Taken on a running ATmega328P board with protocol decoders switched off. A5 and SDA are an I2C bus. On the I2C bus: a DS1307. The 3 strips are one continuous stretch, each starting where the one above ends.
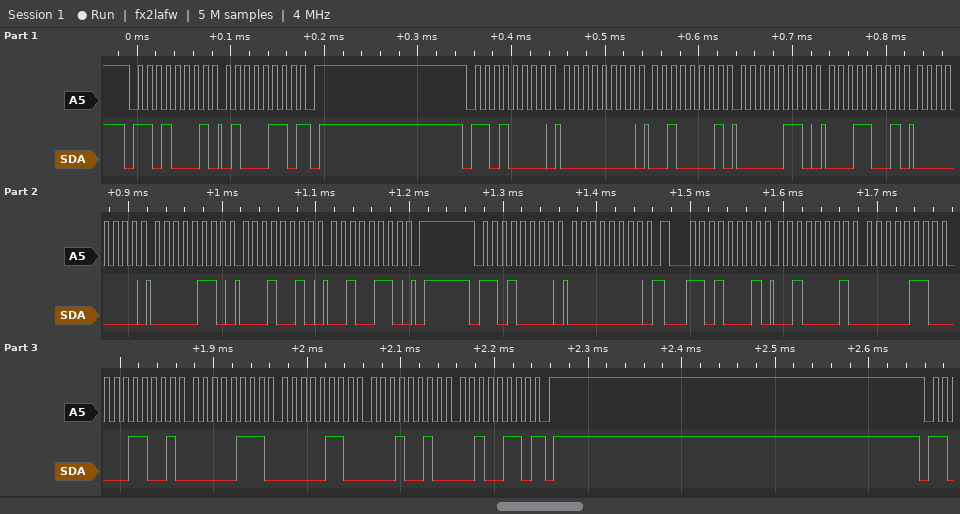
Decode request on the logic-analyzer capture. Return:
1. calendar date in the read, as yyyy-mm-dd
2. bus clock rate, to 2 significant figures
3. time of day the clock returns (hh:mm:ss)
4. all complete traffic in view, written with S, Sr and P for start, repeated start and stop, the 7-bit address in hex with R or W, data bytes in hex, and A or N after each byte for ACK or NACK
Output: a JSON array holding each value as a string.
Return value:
["2026-12-06", "100 kHz", "19:06:21", "S 68R A 46 N P S 68W A 00 A 21 A 06 A 19 A 00 A 06 A 12 A 26 A P S 68W A 00 A Sr 68R A 21 A 06 A 19 A 07 A 06 A 12 A 26 N P"]
